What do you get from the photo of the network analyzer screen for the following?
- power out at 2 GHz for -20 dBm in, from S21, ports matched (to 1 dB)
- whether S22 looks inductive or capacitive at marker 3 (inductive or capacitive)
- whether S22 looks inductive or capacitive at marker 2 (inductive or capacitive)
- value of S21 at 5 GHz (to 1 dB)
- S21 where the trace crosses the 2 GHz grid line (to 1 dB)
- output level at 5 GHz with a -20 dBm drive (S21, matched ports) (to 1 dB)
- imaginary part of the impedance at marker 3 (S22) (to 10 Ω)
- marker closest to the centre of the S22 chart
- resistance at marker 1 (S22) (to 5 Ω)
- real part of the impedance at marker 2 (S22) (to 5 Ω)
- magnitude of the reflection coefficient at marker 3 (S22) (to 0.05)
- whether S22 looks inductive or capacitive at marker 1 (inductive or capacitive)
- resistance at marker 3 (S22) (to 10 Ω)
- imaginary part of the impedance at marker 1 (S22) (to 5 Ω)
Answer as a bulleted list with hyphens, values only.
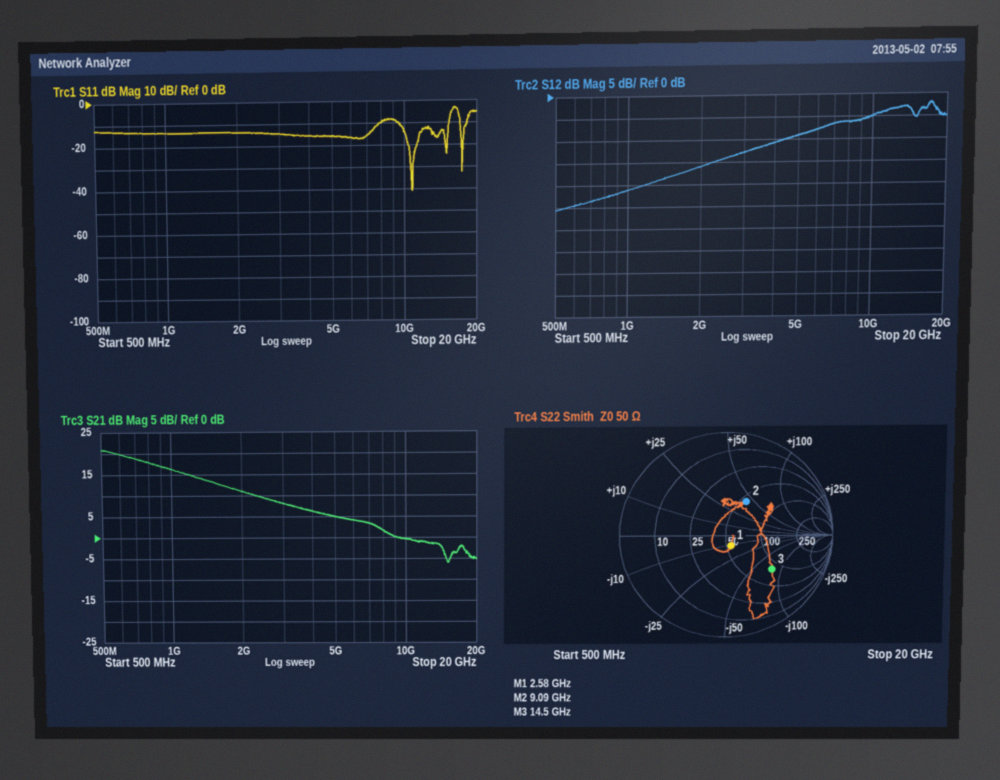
- -9 dBm
- capacitive
- inductive
- 5 dB
- 11 dB
- -15 dBm
- -80 Ω
- marker 1
- 55 Ω
- 55 Ω
- 0.55
- capacitive
- 80 Ω
- -10 Ω
